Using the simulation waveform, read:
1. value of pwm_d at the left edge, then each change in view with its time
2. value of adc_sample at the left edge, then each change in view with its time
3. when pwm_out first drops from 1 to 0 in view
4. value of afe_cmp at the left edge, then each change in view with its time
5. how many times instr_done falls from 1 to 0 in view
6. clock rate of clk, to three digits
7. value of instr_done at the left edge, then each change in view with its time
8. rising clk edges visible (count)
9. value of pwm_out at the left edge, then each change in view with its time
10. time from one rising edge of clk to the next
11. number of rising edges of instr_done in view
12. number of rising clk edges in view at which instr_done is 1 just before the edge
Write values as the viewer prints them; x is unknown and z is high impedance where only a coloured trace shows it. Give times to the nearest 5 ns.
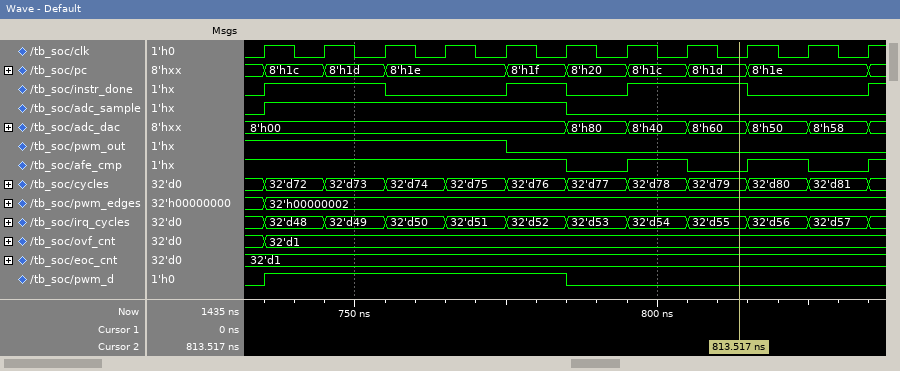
0, 1 at 735 ns, 0 at 785 ns
0, 1 at 735 ns, 0 at 785 ns
775 ns
1, 0 at 785 ns, 1 at 795 ns, 0 at 805 ns, 1 at 815 ns, 0 at 825 ns, 1 at 835 ns
3
100 MHz
0, 1 at 735 ns, 0 at 755 ns, 1 at 775 ns, 0 at 785 ns, 1 at 795 ns, 0 at 815 ns, 1 at 835 ns
11
1, 0 at 775 ns
10 ns
4
5
